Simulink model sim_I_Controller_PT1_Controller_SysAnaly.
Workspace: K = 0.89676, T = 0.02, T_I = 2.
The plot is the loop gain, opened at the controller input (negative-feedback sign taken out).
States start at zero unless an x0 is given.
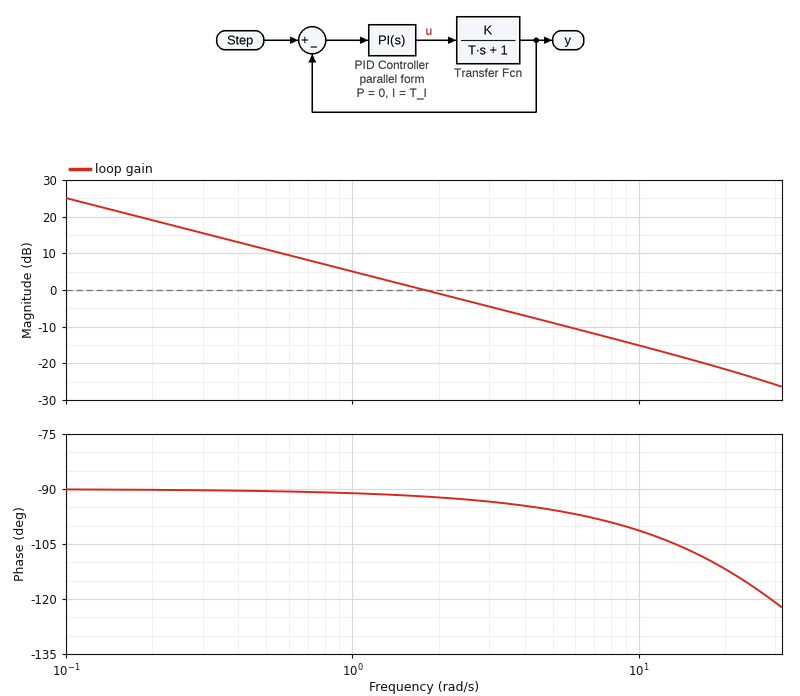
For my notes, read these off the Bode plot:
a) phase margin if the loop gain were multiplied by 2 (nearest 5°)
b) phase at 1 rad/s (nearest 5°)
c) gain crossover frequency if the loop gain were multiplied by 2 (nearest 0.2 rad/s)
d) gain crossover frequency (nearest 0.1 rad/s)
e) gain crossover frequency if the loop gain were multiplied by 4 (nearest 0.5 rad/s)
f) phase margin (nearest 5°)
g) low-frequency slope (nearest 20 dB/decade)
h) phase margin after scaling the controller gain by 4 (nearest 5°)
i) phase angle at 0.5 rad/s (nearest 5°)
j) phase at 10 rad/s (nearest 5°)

85°
-90°
3.6 rad/s
1.8 rad/s
7.0 rad/s
90°
-20 dB/decade
80°
-90°
-100°
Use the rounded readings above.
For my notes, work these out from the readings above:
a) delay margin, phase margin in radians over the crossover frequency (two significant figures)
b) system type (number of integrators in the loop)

0.87 s
1
